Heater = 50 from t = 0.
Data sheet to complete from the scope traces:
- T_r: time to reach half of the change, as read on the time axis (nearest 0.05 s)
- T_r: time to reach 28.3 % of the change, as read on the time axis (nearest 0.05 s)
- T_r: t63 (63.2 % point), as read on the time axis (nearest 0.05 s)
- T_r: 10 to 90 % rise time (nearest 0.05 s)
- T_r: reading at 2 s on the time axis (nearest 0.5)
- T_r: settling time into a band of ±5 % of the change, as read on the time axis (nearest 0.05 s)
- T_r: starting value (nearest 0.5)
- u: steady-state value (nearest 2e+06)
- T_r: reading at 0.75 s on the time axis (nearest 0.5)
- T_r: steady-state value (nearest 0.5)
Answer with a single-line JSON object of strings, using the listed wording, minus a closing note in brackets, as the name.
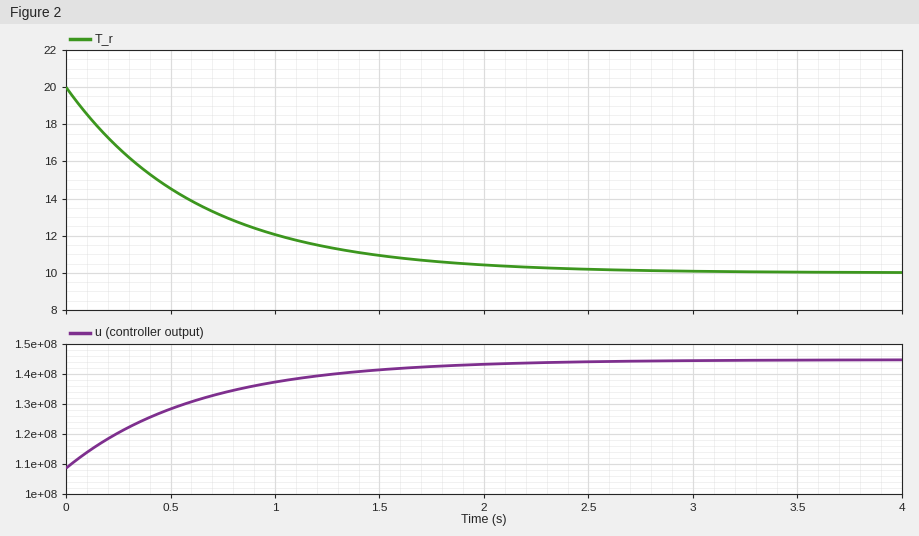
{"T_r: time to reach half of the change, as read on the time axis": "0.45 s", "T_r: time to reach 28.3 % of the change, as read on the time axis": "0.20 s", "T_r: t63 (63.2 % point), as read on the time axis": "0.65 s", "T_r: 10 to 90 % rise time": "1.40 s", "T_r: reading at 2 s on the time axis": "10.5", "T_r: settling time into a band of ±5 % of the change, as read on the time axis": "1.90 s", "T_r: starting value": "20.0", "u: steady-state value": "144000000", "T_r: reading at 0.75 s on the time axis": "13.0", "T_r: steady-state value": "10.0"}
